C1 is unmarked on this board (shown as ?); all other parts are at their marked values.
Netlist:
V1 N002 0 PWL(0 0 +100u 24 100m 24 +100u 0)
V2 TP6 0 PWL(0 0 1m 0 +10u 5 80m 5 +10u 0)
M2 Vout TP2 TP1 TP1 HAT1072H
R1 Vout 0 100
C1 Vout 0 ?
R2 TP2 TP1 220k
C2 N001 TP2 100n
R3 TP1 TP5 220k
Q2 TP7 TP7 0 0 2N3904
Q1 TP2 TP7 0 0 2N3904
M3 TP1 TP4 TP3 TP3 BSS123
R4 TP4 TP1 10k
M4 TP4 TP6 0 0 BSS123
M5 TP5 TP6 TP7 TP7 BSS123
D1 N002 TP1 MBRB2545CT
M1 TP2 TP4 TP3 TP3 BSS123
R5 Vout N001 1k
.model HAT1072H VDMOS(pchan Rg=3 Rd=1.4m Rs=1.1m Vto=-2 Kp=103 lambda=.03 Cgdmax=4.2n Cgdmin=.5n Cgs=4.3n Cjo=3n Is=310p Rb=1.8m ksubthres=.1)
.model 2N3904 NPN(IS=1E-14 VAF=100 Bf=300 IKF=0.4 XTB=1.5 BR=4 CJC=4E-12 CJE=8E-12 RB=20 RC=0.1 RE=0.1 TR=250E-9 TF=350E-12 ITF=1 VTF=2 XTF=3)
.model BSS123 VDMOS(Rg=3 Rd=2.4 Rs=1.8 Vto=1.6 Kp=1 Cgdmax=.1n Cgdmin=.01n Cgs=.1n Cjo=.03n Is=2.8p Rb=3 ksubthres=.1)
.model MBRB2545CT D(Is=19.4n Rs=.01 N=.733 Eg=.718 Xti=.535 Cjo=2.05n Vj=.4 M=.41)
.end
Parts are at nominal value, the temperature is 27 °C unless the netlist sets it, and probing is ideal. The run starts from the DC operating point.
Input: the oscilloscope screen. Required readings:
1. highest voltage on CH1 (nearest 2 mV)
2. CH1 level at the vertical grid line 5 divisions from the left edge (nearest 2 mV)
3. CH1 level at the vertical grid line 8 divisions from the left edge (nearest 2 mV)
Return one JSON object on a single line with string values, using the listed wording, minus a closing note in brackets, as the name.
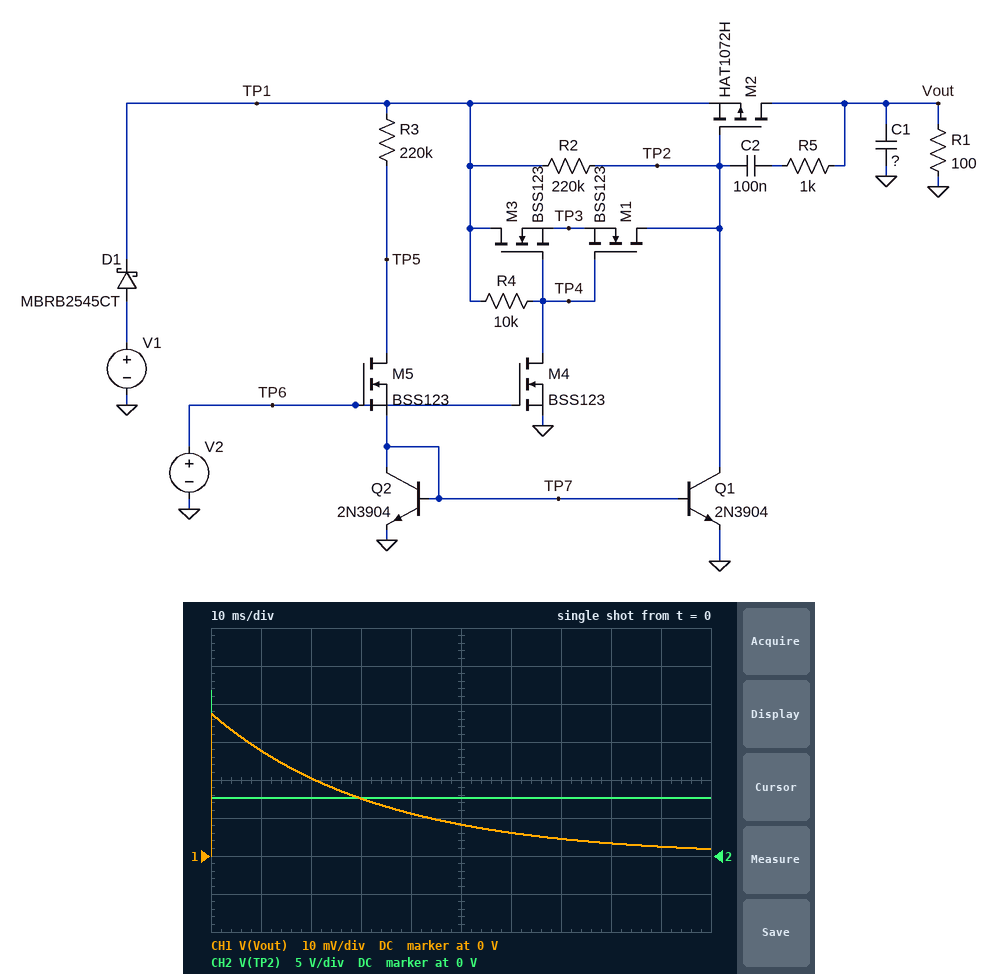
{"highest voltage on CH1": "38 mV", "CH1 level at the vertical grid line 5 divisions from the left edge": "8 mV", "CH1 level at the vertical grid line 8 divisions from the left edge": "4 mV"}
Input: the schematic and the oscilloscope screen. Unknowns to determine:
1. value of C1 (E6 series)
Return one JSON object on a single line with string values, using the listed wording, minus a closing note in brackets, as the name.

{"value of C1": "330 µF"}
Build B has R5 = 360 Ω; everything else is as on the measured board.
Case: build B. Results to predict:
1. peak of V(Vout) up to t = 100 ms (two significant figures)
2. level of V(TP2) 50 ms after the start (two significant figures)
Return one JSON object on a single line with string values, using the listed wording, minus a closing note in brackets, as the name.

{"peak of V(Vout) up to t = 100 ms": "120 mV", "level of V(TP2) 50 ms after the start": "14 V"}
